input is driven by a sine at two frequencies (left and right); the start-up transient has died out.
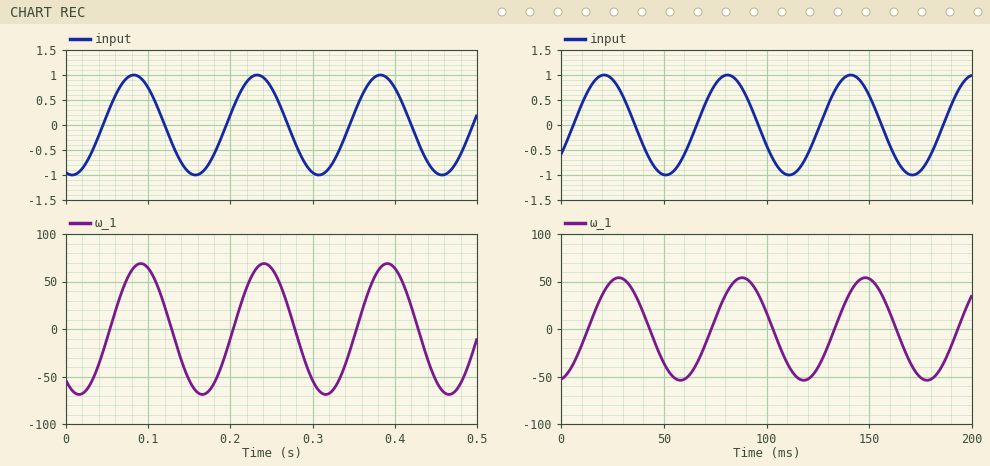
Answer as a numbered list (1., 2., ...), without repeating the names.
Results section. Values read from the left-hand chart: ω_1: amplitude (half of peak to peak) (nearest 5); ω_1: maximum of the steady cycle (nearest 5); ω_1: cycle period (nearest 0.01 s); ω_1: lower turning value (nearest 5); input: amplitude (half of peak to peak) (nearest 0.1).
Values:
1. 70
2. 70
3. 0.15 s
4. -70
5. 1.0
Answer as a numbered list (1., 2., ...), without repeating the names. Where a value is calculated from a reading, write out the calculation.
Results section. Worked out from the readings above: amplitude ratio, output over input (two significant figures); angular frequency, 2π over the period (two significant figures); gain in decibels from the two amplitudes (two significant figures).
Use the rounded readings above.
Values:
1. 70 / 1 = 70
2. 2π / 0.15 = 42 rad/s
3. 20 log10(70 / 1) = 37 dB
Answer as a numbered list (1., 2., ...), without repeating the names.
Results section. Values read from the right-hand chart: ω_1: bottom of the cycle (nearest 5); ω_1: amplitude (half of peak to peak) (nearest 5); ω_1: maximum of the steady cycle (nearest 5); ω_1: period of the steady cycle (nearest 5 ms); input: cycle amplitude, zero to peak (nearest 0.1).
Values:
1. -55
2. 55
3. 55
4. 60 ms
5. 1.0
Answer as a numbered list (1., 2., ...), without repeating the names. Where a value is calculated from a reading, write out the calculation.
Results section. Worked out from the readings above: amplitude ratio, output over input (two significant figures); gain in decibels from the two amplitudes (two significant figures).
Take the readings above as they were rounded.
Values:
1. 55 / 1 = 55
2. 20 log10(55 / 1) = 35 dB
